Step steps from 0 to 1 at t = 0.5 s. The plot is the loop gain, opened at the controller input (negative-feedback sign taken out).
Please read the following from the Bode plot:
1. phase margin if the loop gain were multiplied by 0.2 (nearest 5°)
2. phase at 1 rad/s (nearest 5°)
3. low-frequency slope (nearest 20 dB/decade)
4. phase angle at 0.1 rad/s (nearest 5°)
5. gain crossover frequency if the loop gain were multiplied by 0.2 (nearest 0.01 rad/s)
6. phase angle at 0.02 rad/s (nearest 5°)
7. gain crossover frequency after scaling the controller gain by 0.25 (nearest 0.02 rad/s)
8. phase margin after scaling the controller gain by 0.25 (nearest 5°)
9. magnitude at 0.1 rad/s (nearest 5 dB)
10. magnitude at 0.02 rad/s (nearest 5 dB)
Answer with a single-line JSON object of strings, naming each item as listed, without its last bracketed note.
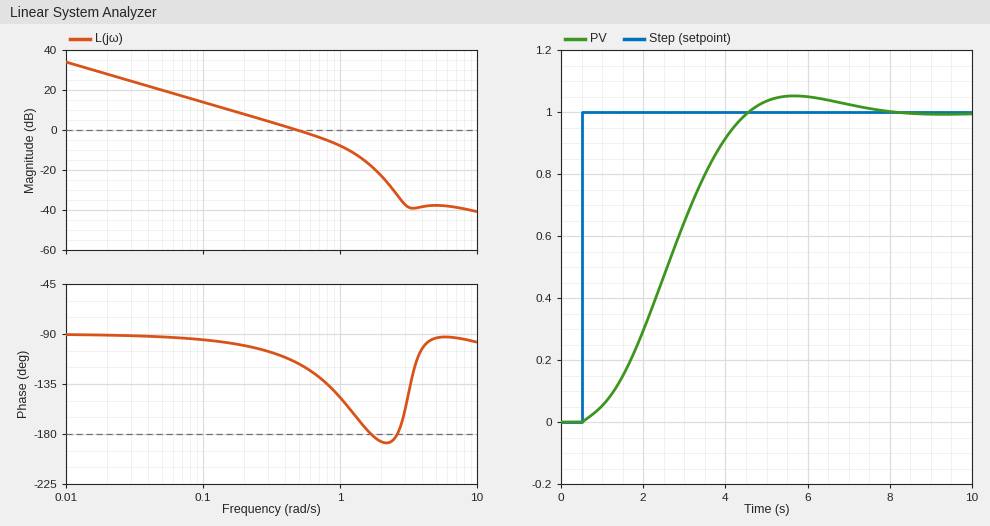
{"phase margin if the loop gain were multiplied by 0.2": "85°", "phase at 1 rad/s": "-145°", "low-frequency slope": "-20 dB/decade", "phase angle at 0.1 rad/s": "-95°", "gain crossover frequency if the loop gain were multiplied by 0.2": "0.10 rad/s", "phase angle at 0.02 rad/s": "-90°", "gain crossover frequency after scaling the controller gain by 0.25": "0.12 rad/s", "phase margin after scaling the controller gain by 0.25": "85°", "magnitude at 0.1 rad/s": "15 dB", "magnitude at 0.02 rad/s": "30 dB"}
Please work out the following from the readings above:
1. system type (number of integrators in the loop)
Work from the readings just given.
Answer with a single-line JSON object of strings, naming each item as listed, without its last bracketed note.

{"system type": "1"}
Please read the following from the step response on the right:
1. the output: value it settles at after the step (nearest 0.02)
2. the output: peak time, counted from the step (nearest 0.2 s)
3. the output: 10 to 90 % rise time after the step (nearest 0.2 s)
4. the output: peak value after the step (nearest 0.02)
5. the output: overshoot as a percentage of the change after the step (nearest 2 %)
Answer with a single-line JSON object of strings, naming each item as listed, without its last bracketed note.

{"the output: value it settles at after the step": "1.00", "the output: peak time, counted from the step": "5.2 s", "the output: 10 to 90 % rise time after the step": "2.6 s", "the output: peak value after the step": "1.06", "the output: overshoot as a percentage of the change after the step": "6 %"}
